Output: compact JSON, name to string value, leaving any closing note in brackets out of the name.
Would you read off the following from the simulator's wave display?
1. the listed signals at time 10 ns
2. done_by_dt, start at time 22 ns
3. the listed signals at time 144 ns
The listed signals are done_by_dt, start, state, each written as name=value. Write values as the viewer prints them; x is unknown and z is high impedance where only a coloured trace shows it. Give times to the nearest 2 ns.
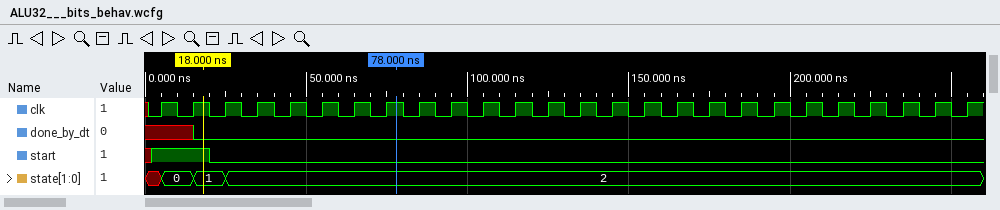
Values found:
{"the listed signals at time 10 ns": "done_by_dt=x, start=1, state=0", "done_by_dt, start at time 22 ns": "done_by_dt=0, start=0", "the listed signals at time 144 ns": "done_by_dt=0, start=0, state=2"}
